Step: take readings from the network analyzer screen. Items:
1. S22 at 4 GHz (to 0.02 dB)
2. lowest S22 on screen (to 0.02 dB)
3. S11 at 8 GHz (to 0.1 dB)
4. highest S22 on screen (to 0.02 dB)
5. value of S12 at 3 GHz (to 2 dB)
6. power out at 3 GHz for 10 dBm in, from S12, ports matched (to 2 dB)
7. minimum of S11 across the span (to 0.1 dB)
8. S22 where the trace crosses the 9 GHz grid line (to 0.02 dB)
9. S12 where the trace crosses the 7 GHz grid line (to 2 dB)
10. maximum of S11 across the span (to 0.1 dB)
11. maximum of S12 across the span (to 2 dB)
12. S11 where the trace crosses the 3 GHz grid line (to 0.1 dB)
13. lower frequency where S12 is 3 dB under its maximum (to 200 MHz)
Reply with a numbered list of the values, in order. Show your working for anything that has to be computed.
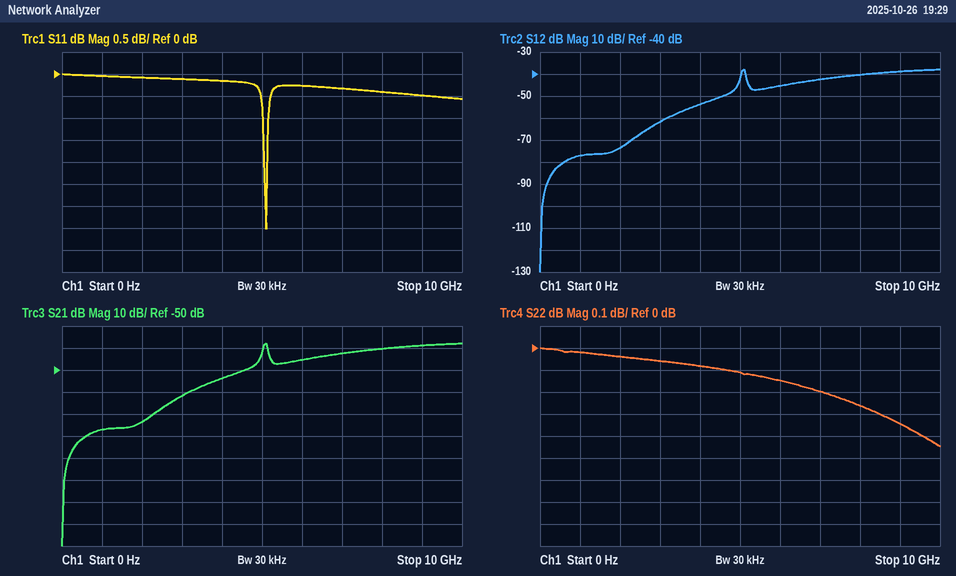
1. -0.08 dB
2. -0.44 dB
3. -0.4 dB
4. 0.00 dB
5. -62 dB
6. 10 dBm + (-62 dB) = -52 dBm
7. -3.5 dB
8. -0.34 dB
9. -42 dB
10. 0.0 dB
11. -38 dB
12. -0.1 dB
13. 5.0 GHz
